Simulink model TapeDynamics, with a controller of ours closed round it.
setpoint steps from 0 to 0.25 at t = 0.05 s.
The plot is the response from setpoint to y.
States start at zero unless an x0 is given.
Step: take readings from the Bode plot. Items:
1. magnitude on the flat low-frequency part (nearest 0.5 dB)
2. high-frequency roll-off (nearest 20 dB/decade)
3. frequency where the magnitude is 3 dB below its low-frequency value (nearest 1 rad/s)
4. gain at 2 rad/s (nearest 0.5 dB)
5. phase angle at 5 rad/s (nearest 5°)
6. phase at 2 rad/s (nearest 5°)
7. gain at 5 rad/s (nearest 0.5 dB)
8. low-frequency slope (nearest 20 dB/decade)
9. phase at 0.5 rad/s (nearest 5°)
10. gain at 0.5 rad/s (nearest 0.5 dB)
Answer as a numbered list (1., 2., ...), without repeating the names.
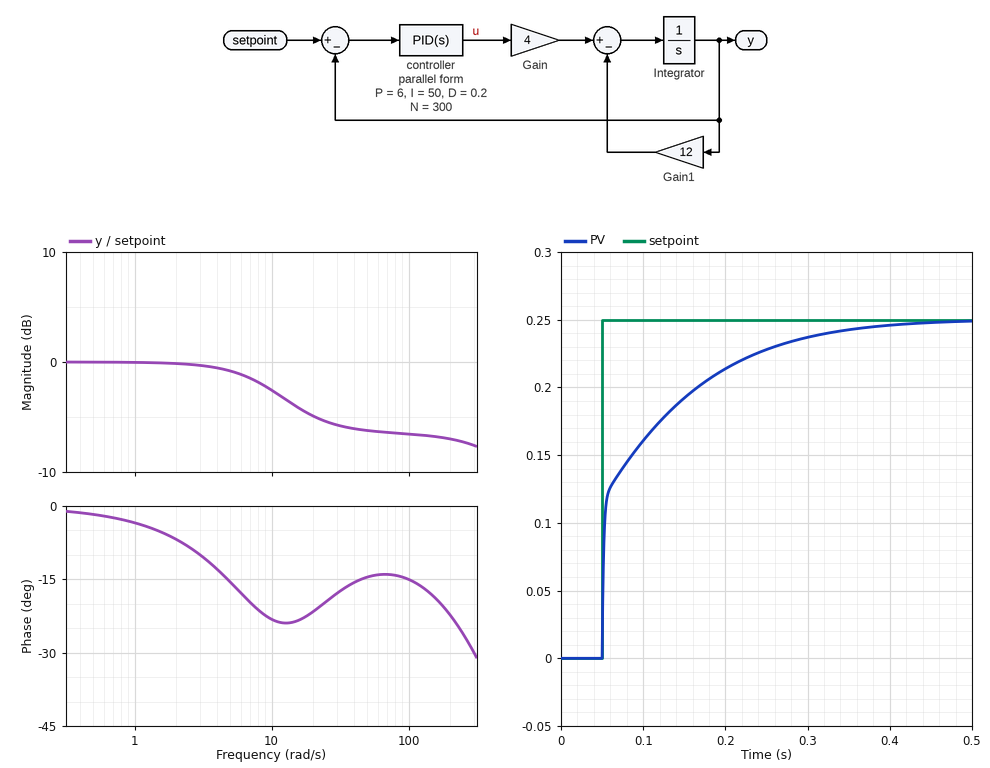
1. 0.0 dB
2. 0 dB/decade
3. 11 rad/s
4. 0.0 dB
5. -15°
6. -5°
7. -1.0 dB
8. 0 dB/decade
9. 0°
10. 0.0 dB
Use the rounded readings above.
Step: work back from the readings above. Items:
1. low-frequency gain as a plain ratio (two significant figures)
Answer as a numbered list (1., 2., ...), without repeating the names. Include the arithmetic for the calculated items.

1. 10^(0 / 20) = 1.0
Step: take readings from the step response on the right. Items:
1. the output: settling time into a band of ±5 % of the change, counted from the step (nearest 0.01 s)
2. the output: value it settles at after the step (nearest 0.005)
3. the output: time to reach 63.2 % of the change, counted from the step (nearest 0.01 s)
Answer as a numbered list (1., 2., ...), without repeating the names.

1. 0.25 s
2. 0.250
3. 0.05 s
